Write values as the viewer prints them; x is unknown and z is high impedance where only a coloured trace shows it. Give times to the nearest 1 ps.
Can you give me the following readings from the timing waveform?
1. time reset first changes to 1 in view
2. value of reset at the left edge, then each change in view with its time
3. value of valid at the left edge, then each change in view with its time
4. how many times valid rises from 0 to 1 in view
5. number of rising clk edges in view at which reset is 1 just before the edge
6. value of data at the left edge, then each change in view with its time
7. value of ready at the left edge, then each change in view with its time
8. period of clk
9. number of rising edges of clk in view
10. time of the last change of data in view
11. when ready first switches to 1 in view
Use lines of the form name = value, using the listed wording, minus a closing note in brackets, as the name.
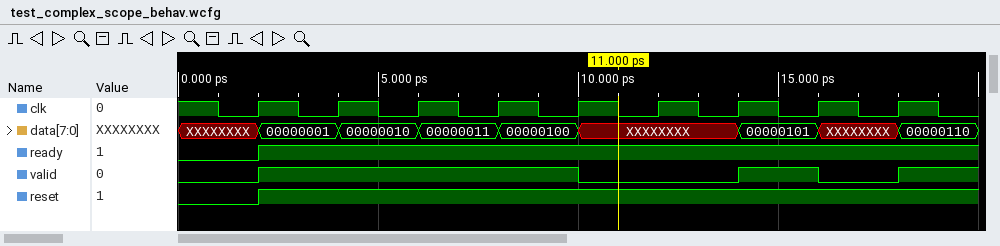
time reset first changes to 1 in view = 2 ps
value of reset at the left edge, then each change in view with its time = 0, 1 at 2 ps
value of valid at the left edge, then each change in view with its time = 0, 1 at 2 ps, 0 at 10 ps, 1 at 14 ps, 0 at 16 ps, 1 at 18 ps
how many times valid rises from 0 to 1 in view = 3
number of rising clk edges in view at which reset is 1 just before the edge = 8
value of data at the left edge, then each change in view with its time = XXXXXXXX, 00000001 at 2 ps, 00000010 at 4 ps, 00000011 at 6 ps, 00000100 at 8 ps, XXXXXXXX at 10 ps, 00000101 at 14 ps, XXXXXXXX at 16 ps, 00000110 at 18 ps
value of ready at the left edge, then each change in view with its time = 0, 1 at 2 ps
period of clk = 2 ps
number of rising edges of clk in view = 9
time of the last change of data in view = 18 ps
when ready first switches to 1 in view = 2 ps
